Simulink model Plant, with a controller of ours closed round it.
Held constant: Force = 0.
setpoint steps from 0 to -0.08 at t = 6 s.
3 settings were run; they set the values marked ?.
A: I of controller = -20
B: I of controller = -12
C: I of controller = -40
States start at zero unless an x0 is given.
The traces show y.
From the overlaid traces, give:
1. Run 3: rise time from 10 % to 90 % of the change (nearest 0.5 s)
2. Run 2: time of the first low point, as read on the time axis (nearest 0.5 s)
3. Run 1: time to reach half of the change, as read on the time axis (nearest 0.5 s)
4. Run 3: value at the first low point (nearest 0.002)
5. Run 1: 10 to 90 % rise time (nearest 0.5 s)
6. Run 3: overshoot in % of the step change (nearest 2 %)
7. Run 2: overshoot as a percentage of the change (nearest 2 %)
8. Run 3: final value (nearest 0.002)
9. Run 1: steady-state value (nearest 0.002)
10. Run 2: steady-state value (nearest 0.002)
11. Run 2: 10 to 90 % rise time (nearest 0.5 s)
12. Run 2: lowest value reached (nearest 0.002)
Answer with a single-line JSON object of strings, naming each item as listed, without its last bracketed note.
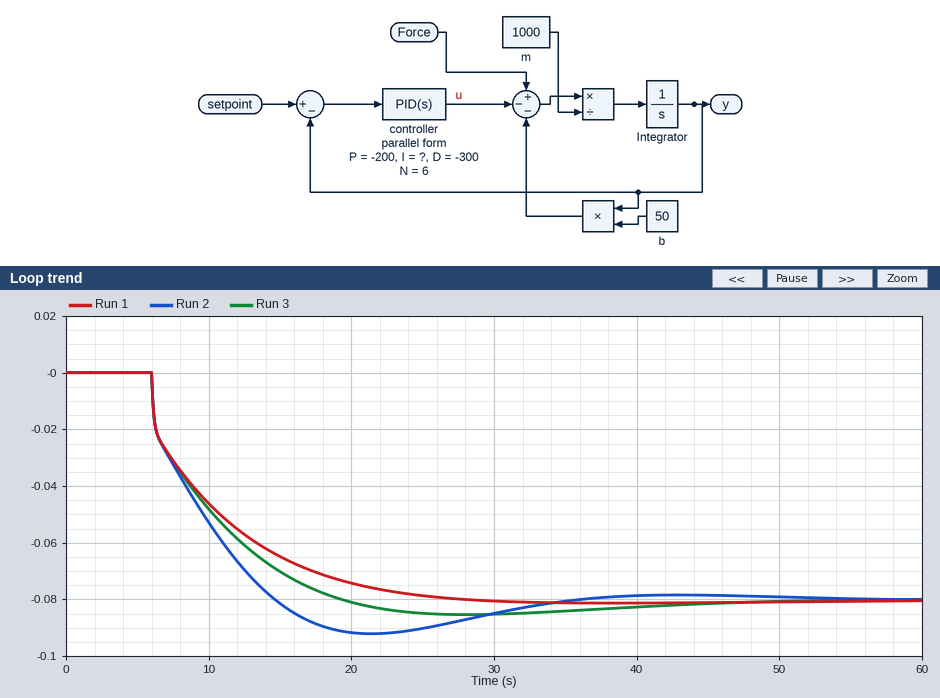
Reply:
{"Run 3: rise time from 10 % to 90 % of the change": "9.5 s", "Run 2: time of the first low point, as read on the time axis": "21.5 s", "Run 1: time to reach half of the change, as read on the time axis": "9.0 s", "Run 3: value at the first low point": "-0.086", "Run 1: 10 to 90 % rise time": "12.5 s", "Run 3: overshoot in % of the step change": "6 %", "Run 2: overshoot as a percentage of the change": "16 %", "Run 3: final value": "-0.080", "Run 1: steady-state value": "-0.080", "Run 2: steady-state value": "-0.080", "Run 2: 10 to 90 % rise time": "7.0 s", "Run 2: lowest value reached": "-0.092"}
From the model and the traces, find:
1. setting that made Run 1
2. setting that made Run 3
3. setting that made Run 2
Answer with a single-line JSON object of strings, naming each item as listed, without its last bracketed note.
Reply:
{"setting that made Run 1": "B", "setting that made Run 3": "A", "setting that made Run 2": "C"}
